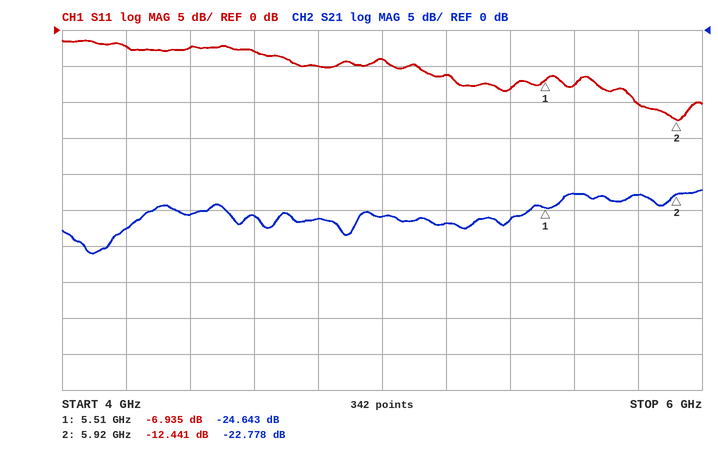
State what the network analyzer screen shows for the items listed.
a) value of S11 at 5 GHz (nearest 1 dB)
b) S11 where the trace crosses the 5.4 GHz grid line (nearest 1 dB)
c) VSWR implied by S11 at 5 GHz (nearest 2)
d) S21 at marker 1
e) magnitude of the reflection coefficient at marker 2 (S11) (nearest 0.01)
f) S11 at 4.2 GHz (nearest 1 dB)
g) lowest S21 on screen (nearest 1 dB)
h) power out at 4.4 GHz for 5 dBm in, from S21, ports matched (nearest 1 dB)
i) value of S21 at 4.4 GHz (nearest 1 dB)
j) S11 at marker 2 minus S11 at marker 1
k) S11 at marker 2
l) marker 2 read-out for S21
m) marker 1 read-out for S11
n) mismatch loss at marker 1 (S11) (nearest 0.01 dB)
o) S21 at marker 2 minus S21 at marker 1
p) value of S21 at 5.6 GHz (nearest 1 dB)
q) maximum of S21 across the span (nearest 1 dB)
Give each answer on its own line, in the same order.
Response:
-4 dB
-8 dB
4
-24.643 dB
0.24
-2 dB
-31 dB
-21 dBm
-26 dB
-5.506 dB
-12.441 dB
-22.778 dB
-6.935 dB
0.98 dB
1.865 dB
-23 dB
-22 dB
